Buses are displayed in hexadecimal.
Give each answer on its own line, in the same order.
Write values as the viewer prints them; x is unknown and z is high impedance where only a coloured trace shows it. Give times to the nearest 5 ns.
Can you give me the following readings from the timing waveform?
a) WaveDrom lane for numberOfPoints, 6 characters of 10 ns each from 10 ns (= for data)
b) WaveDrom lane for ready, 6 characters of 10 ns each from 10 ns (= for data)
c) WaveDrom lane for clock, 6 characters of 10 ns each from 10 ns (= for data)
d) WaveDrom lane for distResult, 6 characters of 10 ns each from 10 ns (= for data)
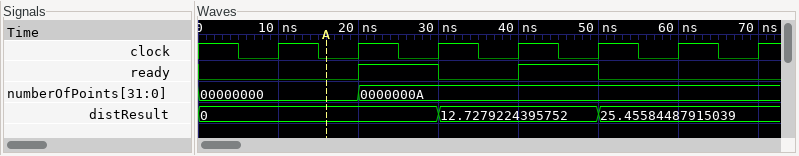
{name: 'numberOfPoints', wave: '==....', data: '00000000 0000000A'}
{name: 'ready', wave: '01010.'}
{name: 'clock', wave: 'p.....'}
{name: 'distResult', wave: '=.=.=.', data: '0 12.7279224395752 25.45584487915039'}
